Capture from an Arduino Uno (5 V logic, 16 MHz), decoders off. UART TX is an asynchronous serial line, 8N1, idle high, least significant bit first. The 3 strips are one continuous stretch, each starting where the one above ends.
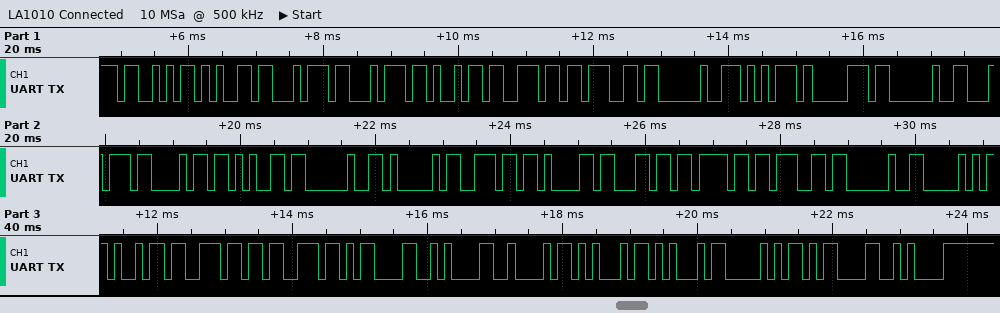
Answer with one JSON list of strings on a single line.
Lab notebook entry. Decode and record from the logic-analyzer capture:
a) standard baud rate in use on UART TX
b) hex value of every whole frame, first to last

["9600 baud", "53 65 74 74 69 6E 67 20 75 70 20 74 68 65 20 41 6E 61 6C 6F 67 20 50 69 6E 73 0D 0A 42 45 45 50 0D 0A"]
